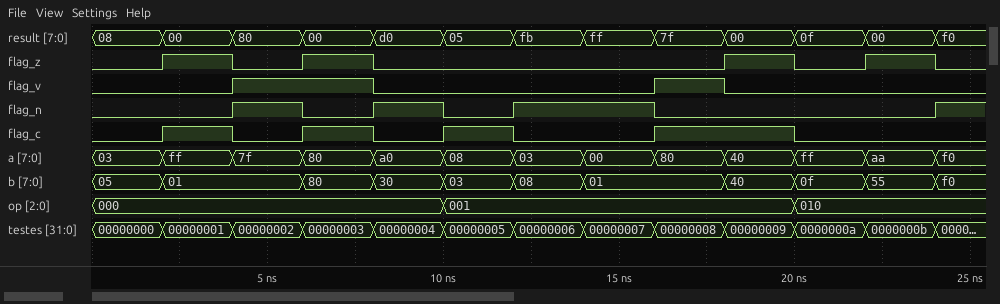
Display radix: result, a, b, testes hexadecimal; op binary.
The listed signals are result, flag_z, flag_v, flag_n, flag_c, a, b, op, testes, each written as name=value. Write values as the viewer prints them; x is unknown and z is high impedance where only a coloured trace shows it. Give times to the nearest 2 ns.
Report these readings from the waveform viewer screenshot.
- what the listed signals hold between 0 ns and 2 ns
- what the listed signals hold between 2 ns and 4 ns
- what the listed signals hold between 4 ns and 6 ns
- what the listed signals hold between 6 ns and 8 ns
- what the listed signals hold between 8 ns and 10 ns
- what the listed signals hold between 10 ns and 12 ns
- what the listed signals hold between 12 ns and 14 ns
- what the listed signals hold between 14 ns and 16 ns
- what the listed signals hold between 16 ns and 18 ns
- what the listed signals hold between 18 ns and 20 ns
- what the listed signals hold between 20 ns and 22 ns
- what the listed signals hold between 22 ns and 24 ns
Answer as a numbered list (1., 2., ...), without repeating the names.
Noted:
1. result=08, flag_z=0, flag_v=0, flag_n=0, flag_c=0, a=03, b=05, op=000, testes=00000000
2. result=00, flag_z=1, flag_v=0, flag_n=0, flag_c=1, a=ff, b=01, op=000, testes=00000001
3. result=80, flag_z=0, flag_v=1, flag_n=1, flag_c=0, a=7f, b=01, op=000, testes=00000002
4. result=00, flag_z=1, flag_v=1, flag_n=0, flag_c=1, a=80, b=80, op=000, testes=00000003
5. result=d0, flag_z=0, flag_v=0, flag_n=1, flag_c=0, a=a0, b=30, op=000, testes=00000004
6. result=05, flag_z=0, flag_v=0, flag_n=0, flag_c=1, a=08, b=03, op=001, testes=00000005
7. result=fb, flag_z=0, flag_v=0, flag_n=1, flag_c=0, a=03, b=08, op=001, testes=00000006
8. result=ff, flag_z=0, flag_v=0, flag_n=1, flag_c=0, a=00, b=01, op=001, testes=00000007
9. result=7f, flag_z=0, flag_v=1, flag_n=0, flag_c=1, a=80, b=01, op=001, testes=00000008
10. result=00, flag_z=1, flag_v=0, flag_n=0, flag_c=1, a=40, b=40, op=001, testes=00000009
11. result=0f, flag_z=0, flag_v=0, flag_n=0, flag_c=0, a=ff, b=0f, op=010, testes=0000000a
12. result=00, flag_z=1, flag_v=0, flag_n=0, flag_c=0, a=aa, b=55, op=010, testes=0000000b
